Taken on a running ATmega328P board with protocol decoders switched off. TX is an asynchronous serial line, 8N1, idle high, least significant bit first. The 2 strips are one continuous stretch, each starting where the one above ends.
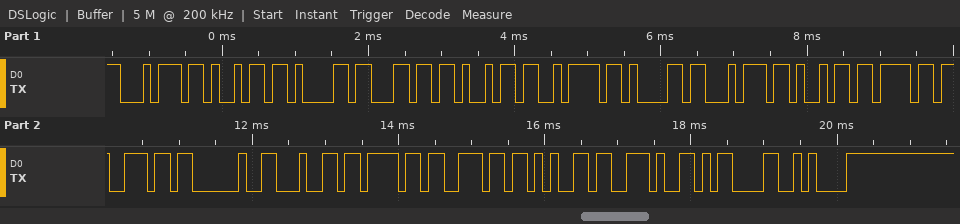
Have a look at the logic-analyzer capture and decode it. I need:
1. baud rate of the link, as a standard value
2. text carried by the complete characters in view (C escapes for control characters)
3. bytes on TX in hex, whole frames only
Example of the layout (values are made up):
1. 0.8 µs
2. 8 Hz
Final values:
1. 9600 baud
2. "tialization done.\r\n"
3. 74 69 61 6C 69 7A 61 74 69 6F 6E 20 64 6F 6E 65 2E 0D 0A
